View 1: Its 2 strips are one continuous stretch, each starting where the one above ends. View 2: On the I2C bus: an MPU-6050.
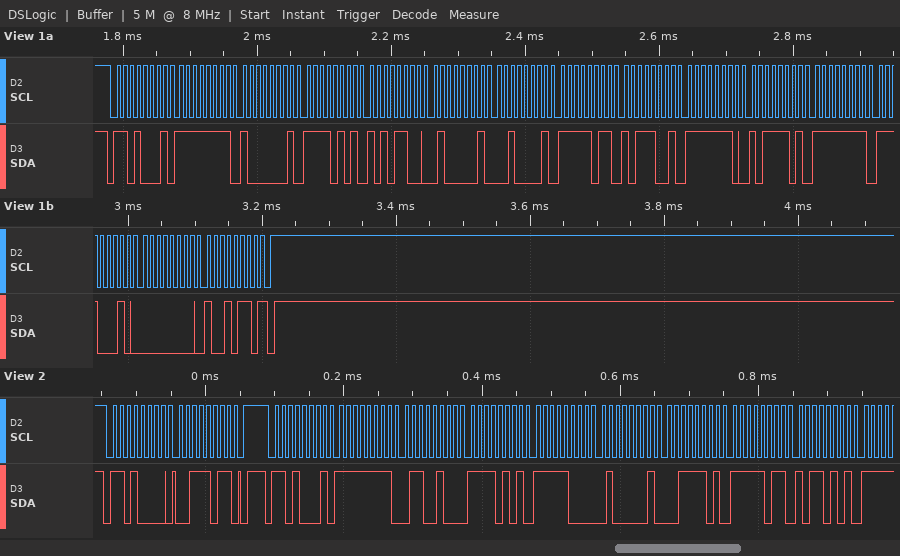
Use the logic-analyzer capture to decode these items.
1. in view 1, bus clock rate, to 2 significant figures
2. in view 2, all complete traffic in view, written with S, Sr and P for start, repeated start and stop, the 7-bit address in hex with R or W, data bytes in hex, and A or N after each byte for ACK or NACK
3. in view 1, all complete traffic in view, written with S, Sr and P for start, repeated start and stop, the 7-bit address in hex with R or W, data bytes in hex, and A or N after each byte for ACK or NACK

100 kHz
S 68W A 3B A P S 68R A FF A 64 A F5 A F8 A 41 A 3D A FB A B5 A
S 68R A FF A 81 A F5 A AC A 41 A 21 A FB A B9 A FE A BD A FF A E2 A 00 A 96 N P
